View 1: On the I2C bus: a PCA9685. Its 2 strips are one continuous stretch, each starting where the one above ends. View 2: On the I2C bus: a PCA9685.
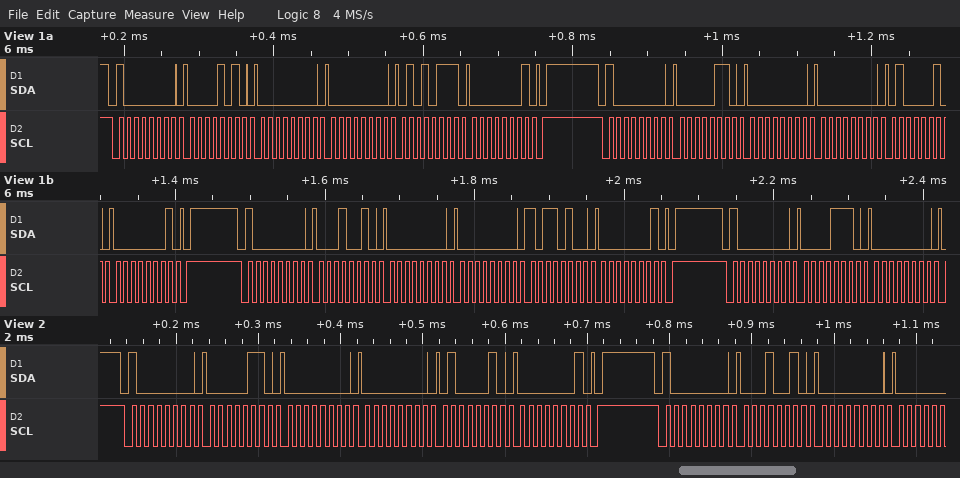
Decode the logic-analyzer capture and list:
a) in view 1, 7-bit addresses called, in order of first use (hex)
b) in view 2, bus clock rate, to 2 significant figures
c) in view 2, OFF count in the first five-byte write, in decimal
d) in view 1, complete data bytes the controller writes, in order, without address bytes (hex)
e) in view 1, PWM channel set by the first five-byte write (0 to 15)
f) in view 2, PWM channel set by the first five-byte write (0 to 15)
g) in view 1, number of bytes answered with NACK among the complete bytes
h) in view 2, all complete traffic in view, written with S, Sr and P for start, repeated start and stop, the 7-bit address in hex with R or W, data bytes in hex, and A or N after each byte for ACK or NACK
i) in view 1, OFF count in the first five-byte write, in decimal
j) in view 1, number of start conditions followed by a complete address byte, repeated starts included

0x40
100 kHz
322
0A 00 00 57 01 06 00 00 42 01 12 00 00 B4 01 0E 00
1
0
0
S 40W A 06 A 00 A 00 A 42 A 01 A P S 40W A 12 A 00 A
343
4
